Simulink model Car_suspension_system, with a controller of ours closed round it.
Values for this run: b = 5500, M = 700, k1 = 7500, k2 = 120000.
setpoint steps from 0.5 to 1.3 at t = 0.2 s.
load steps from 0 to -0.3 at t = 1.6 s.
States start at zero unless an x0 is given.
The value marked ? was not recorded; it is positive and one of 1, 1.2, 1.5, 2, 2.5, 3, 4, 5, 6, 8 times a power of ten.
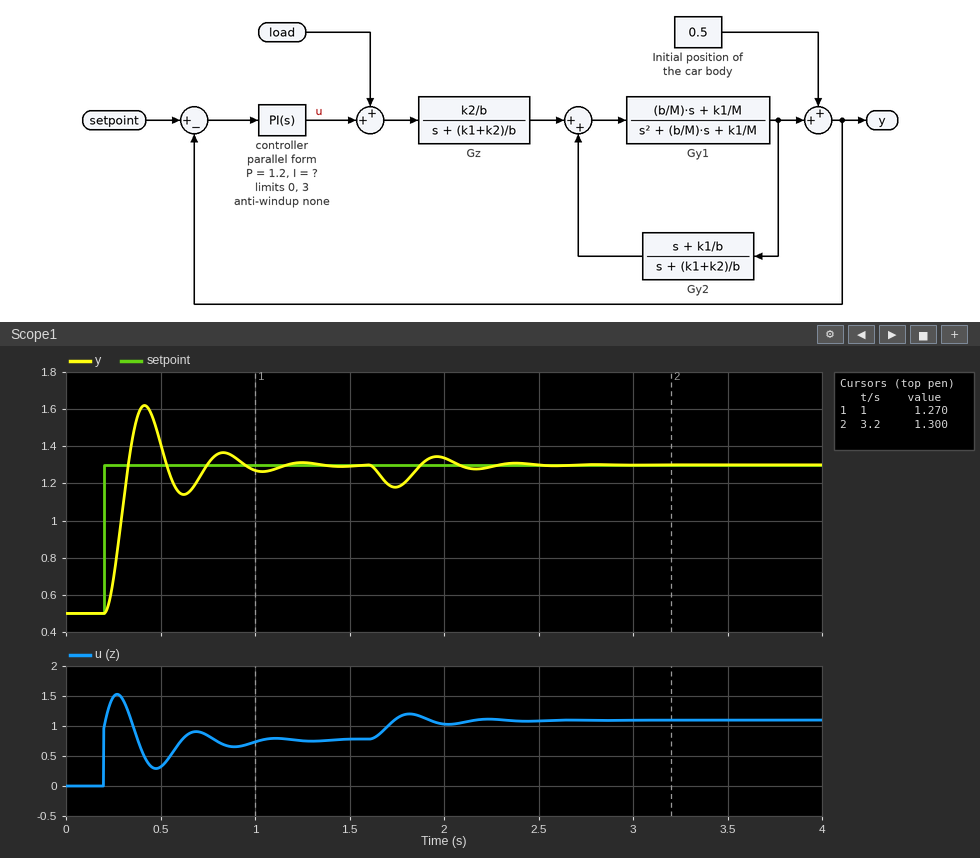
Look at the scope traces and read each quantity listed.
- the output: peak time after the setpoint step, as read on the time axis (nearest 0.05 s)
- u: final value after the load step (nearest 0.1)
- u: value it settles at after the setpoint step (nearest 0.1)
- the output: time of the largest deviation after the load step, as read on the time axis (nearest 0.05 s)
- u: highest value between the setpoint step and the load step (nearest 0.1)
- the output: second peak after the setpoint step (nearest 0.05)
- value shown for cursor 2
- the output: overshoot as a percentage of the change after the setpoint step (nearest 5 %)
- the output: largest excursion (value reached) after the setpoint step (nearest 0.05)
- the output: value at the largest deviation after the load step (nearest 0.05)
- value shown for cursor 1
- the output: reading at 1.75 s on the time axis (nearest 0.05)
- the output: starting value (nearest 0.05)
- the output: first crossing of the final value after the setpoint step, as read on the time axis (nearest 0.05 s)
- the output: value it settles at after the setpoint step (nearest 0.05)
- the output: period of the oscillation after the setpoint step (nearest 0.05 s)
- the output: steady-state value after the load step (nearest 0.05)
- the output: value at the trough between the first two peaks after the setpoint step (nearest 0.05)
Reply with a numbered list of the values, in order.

1. 0.40 s
2. 1.1
3. 0.8
4. 1.75 s
5. 1.5
6. 1.35
7. 1.300
8. 40 %
9. 1.60
10. 1.20
11. 1.270
12. 1.20
13. 0.50
14. 0.35 s
15. 1.30
16. 0.40 s
17. 1.30
18. 1.15
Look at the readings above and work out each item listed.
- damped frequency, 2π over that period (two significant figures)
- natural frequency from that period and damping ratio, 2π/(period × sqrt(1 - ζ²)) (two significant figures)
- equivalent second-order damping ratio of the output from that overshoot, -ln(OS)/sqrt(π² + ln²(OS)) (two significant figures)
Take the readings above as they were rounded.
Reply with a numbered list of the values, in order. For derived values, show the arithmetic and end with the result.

1. 2π / 0.4 = 16 rad/s
2. 2π / (0.4 × sqrt(1 - 0.28²)) = 16 rad/s
3. ln(0.4) = -0.916; 0.916 / sqrt(9.870 + 0.840) = 0.28
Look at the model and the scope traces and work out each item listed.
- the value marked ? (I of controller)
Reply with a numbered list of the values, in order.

1. 20
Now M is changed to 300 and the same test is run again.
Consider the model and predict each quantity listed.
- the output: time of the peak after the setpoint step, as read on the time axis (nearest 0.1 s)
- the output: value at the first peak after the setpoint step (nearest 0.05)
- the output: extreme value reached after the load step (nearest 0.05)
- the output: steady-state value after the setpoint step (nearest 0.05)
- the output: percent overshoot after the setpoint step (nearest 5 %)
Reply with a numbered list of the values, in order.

1. 0.3 s
2. 1.50
3. 1.15
4. 1.30
5. 25 %
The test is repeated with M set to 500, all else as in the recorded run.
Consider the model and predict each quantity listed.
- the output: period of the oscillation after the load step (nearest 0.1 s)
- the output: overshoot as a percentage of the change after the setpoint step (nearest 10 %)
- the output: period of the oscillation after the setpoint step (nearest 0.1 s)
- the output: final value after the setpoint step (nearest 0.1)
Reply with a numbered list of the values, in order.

1. 0.3 s
2. 30 %
3. 0.3 s
4. 1.3
